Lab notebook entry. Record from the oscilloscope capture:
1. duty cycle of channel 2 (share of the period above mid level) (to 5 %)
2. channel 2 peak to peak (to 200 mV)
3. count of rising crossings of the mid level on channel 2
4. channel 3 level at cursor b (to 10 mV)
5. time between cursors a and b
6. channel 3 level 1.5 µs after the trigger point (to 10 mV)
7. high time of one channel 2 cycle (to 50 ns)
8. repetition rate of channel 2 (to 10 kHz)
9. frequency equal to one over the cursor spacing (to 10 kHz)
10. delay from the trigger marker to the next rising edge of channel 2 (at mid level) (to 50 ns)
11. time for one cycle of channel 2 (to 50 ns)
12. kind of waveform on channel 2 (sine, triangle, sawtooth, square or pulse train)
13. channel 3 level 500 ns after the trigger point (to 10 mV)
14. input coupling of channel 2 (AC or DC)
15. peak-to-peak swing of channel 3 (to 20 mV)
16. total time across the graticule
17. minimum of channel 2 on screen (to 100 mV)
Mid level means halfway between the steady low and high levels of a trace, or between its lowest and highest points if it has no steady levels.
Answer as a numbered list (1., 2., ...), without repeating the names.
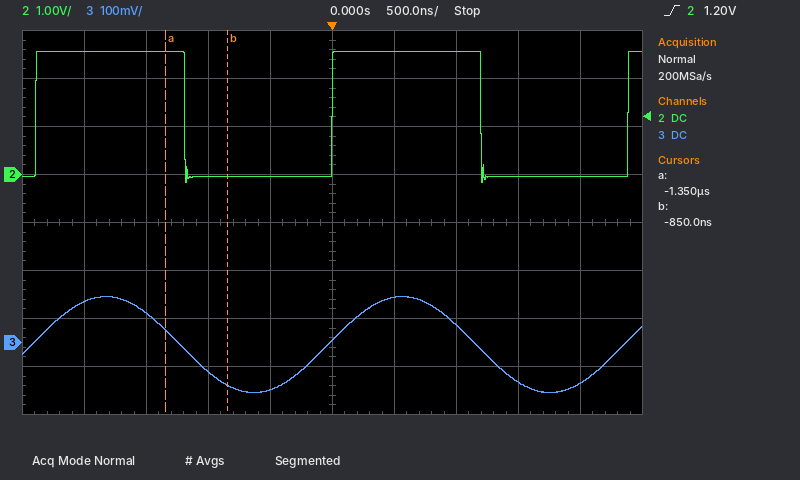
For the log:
1. 50 %
2. 2.8 V
3. 3
4. -90 mV
5. 500 ns
6. -80 mV
7. 1.20 µs
8. 420 kHz
9. 2.00 MHz
10. 2.40 µs
11. 2.40 µs
12. square
13. 90 mV
14. DC
15. 200 mV
16. 5 µs
17. -200 mV
